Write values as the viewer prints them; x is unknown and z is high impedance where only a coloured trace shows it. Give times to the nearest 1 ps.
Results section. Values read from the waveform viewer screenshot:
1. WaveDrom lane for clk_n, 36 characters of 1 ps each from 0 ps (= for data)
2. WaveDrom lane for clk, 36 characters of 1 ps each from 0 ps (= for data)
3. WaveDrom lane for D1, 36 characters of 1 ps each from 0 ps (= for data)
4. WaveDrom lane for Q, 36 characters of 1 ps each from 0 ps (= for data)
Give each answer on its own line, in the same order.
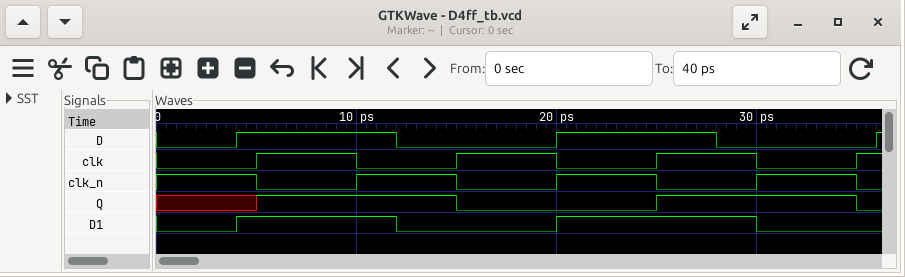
{name: 'clk_n', wave: '1....0....1....0....1....0....1....0'}
{name: 'clk', wave: '0....1....0....1....0....1....0....1'}
{name: 'D1', wave: '0...1.......0.......1.........0.....'}
{name: 'Q', wave: 'x....1.........0.........1.........0'}
